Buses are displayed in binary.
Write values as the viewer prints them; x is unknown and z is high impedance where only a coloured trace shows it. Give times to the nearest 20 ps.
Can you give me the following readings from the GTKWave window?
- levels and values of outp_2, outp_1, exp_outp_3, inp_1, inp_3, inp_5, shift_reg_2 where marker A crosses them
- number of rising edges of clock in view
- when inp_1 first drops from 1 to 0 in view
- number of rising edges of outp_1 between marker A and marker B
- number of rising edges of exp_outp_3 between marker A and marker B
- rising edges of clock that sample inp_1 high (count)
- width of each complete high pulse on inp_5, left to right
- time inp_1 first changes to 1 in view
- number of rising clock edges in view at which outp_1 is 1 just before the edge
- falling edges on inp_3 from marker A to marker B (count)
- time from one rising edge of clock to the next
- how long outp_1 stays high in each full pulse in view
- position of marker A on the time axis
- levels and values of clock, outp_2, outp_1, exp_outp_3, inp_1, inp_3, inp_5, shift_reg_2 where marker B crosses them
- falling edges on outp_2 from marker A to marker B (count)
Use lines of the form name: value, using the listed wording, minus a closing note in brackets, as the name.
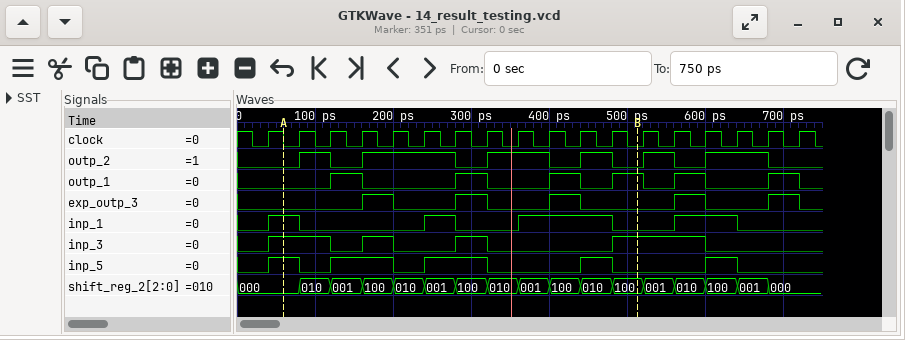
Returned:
levels and values of outp_2, outp_1, exp_outp_3, inp_1, inp_3, inp_5, shift_reg_2 where marker A crosses them: outp_2=0, outp_1=0, exp_outp_3=0, inp_1=1, inp_3=1, inp_5=1, shift_reg_2=000
number of rising edges of clock in view: 18
when inp_1 first drops from 1 to 0 in view: 80 ps
number of rising edges of outp_1 between marker A and marker B: 4
number of rising edges of exp_outp_3 between marker A and marker B: 3
rising edges of clock that sample inp_1 high: 7
width of each complete high pulse on inp_5, left to right: 40 ps, 80 ps, 80 ps, 40 ps, 40 ps
time inp_1 first changes to 1 in view: 40 ps
number of rising clock edges in view at which outp_1 is 1 just before the edge: 6
falling edges on inp_3 from marker A to marker B: 3
time from one rising edge of clock to the next: 40 ps
how long outp_1 stays high in each full pulse in view: 40 ps, 40 ps, 40 ps, 40 ps, 40 ps, 40 ps
position of marker A on the time axis: 60 ps
levels and values of clock, outp_2, outp_1, exp_outp_3, inp_1, inp_3, inp_5, shift_reg_2 where marker B crosses them: clock=0, outp_2=0, outp_1=1, exp_outp_3=0, inp_1=0, inp_3=1, inp_5=0, shift_reg_2=100
falling edges on outp_2 from marker A to marker B: 4
